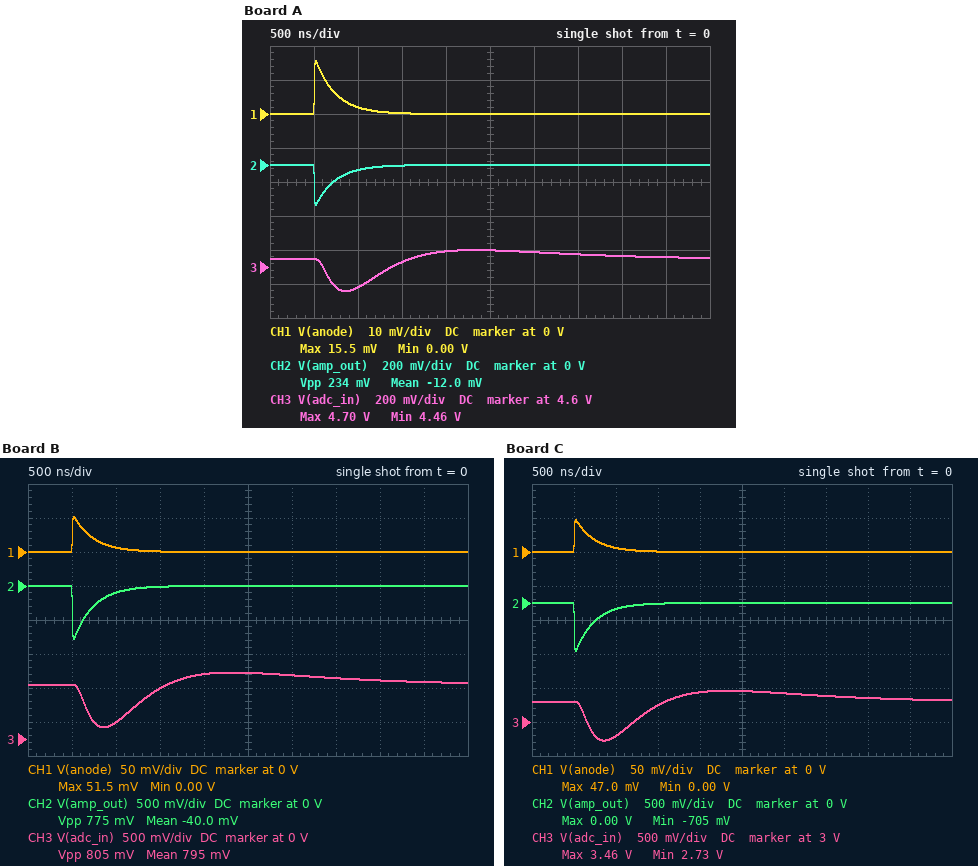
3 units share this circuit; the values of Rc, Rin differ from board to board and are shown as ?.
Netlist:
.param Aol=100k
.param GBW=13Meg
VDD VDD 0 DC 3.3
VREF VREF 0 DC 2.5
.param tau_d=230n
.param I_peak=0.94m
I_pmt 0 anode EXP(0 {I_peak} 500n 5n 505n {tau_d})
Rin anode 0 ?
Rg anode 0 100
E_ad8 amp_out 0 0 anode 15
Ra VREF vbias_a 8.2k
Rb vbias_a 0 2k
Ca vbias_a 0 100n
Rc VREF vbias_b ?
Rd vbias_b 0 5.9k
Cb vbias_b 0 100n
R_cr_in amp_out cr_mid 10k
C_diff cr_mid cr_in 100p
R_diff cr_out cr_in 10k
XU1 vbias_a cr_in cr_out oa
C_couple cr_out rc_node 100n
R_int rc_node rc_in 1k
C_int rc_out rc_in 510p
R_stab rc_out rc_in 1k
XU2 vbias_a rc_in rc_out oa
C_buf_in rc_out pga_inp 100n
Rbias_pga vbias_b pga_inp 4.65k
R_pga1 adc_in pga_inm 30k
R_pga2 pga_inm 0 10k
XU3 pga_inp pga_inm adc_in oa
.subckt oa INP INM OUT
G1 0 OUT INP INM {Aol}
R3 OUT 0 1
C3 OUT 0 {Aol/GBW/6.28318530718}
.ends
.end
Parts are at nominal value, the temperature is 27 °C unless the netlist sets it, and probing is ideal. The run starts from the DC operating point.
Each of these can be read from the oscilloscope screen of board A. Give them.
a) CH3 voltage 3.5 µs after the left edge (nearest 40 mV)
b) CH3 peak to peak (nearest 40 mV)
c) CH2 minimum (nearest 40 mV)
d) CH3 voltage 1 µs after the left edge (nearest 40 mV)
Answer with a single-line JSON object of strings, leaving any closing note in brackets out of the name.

{"CH3 voltage 3.5 µs after the left edge": "4.68 V", "CH3 peak to peak": "240 mV", "CH2 minimum": "-240 mV", "CH3 voltage 1 µs after the left edge": "4.48 V"}
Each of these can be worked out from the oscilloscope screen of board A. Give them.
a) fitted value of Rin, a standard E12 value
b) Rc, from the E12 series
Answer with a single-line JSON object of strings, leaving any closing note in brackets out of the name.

{"fitted value of Rin, a standard E12 value": "22 Ω", "Rc, from the E12 series": "6.8 kΩ"}
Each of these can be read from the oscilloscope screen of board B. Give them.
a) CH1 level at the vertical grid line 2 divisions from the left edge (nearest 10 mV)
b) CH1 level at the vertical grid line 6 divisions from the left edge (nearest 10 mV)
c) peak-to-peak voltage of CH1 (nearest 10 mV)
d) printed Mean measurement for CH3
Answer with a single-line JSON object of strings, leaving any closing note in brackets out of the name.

{"CH1 level at the vertical grid line 2 divisions from the left edge": "10 mV", "CH1 level at the vertical grid line 6 divisions from the left edge": "0 V", "peak-to-peak voltage of CH1": "50 mV", "printed Mean measurement for CH3": "795 mV"}
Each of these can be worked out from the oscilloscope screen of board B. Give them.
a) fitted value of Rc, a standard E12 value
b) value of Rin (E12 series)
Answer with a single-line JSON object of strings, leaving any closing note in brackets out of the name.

{"fitted value of Rc, a standard E12 value": "68 kΩ", "value of Rin": "150 Ω"}
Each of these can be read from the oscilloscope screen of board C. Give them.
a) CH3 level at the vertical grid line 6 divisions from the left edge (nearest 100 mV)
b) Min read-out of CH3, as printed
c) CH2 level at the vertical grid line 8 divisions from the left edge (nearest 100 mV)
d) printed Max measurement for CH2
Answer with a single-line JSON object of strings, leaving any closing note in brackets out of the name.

{"CH3 level at the vertical grid line 6 divisions from the left edge": "3.4 V", "Min read-out of CH3, as printed": "2.73 V", "CH2 level at the vertical grid line 8 divisions from the left edge": "0 V", "printed Max measurement for CH2": "0.00 V"}
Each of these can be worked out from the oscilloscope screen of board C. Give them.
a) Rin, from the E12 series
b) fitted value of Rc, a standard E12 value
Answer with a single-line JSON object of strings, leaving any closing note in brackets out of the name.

{"Rin, from the E12 series": "120 Ω", "fitted value of Rc, a standard E12 value": "12 kΩ"}
